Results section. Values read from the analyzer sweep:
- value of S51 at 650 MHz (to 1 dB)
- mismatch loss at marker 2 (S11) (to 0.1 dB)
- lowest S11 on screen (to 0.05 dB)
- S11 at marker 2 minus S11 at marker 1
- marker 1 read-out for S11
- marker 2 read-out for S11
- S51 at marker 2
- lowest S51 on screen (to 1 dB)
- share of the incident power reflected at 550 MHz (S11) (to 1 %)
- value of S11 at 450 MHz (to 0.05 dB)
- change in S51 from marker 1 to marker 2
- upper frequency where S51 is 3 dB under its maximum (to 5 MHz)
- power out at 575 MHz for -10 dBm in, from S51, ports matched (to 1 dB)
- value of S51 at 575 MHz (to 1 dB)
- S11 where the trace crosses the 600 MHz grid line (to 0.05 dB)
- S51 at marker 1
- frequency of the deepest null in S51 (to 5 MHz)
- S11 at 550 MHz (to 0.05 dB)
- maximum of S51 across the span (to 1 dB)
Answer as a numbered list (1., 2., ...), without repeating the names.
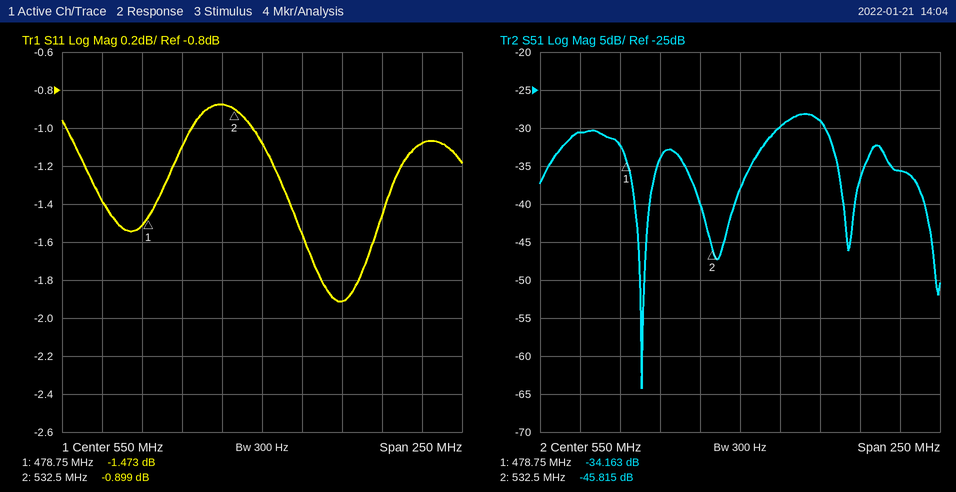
1. -36 dB
2. 7.3 dB
3. -1.90 dB
4. 0.574 dB
5. -1.473 dB
6. -0.899 dB
7. -45.815 dB
8. -64 dB
9. 78 %
10. -1.40 dB
11. -11.652 dB
12. 605 MHz
13. -40 dBm
14. -30 dB
15. -1.90 dB
16. -34.163 dB
17. 490 MHz
18. -1.10 dB
19. -28 dB
